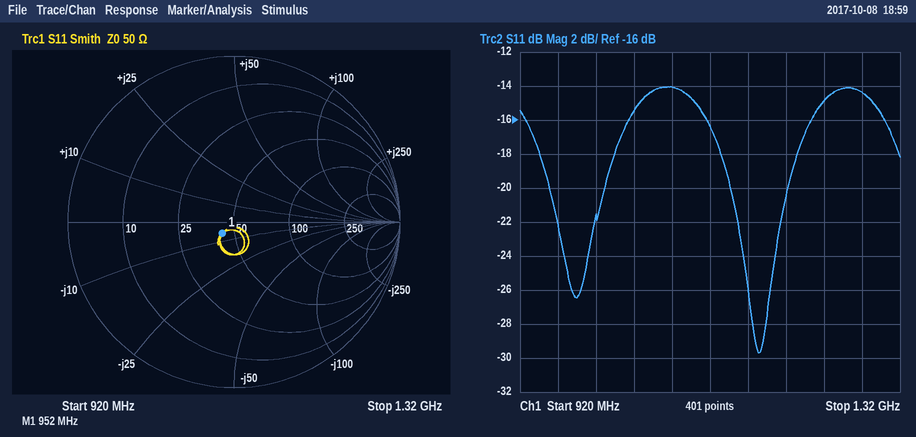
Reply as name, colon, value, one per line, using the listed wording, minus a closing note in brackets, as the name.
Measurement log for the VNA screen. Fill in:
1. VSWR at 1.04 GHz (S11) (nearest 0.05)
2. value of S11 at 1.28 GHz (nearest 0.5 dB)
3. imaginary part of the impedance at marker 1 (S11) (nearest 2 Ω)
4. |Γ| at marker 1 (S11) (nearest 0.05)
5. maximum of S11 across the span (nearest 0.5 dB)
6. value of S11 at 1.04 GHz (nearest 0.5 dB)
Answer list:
VSWR at 1.04 GHz (S11): 1.40
value of S11 at 1.28 GHz: -14.5 dB
imaginary part of the impedance at marker 1 (S11): -6 Ω
|Γ| at marker 1 (S11): 0.10
maximum of S11 across the span: -14.0 dB
value of S11 at 1.04 GHz: -15.5 dB
